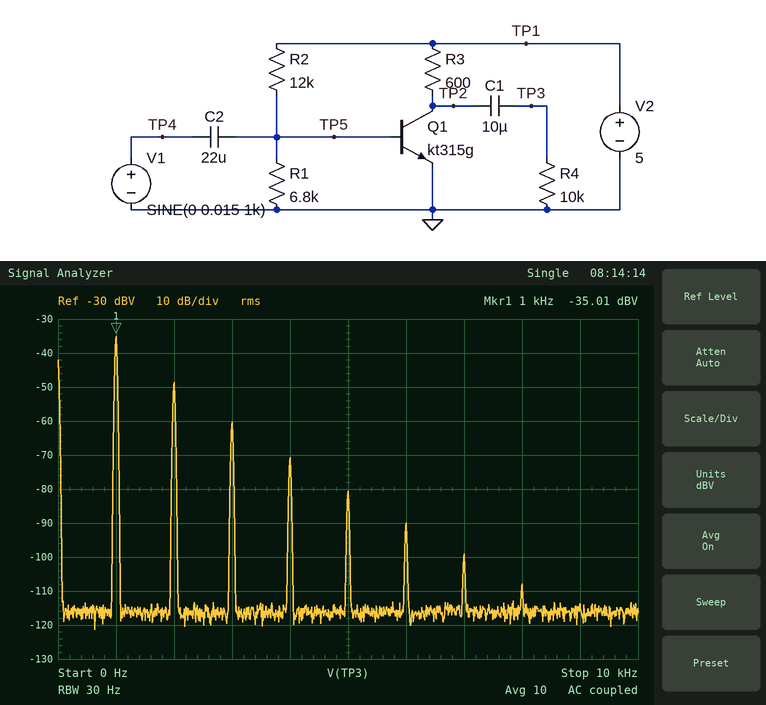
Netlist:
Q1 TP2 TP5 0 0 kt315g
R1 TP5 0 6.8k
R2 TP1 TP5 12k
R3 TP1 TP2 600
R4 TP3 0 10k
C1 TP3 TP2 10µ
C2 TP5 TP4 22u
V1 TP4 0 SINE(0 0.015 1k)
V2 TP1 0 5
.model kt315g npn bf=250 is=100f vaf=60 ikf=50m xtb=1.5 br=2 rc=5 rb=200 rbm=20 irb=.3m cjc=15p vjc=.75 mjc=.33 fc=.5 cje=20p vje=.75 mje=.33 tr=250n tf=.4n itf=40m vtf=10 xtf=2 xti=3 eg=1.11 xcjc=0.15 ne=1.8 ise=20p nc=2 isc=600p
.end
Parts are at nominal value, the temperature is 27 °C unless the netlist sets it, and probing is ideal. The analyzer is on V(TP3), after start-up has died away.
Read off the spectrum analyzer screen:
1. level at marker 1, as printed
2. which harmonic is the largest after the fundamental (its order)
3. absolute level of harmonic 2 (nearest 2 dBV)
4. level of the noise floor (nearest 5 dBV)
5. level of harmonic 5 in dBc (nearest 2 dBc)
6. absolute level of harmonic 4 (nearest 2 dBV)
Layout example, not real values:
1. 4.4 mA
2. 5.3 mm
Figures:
1. -35.01 dBV
2. 2
3. -48 dBV
4. -115 dBV
5. -46 dBc
6. -70 dBV
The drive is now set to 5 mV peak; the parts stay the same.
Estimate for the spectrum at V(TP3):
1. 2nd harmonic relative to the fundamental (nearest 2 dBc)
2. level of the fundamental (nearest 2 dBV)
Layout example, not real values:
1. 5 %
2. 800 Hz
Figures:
1. -24 dBc
2. -46 dBV
